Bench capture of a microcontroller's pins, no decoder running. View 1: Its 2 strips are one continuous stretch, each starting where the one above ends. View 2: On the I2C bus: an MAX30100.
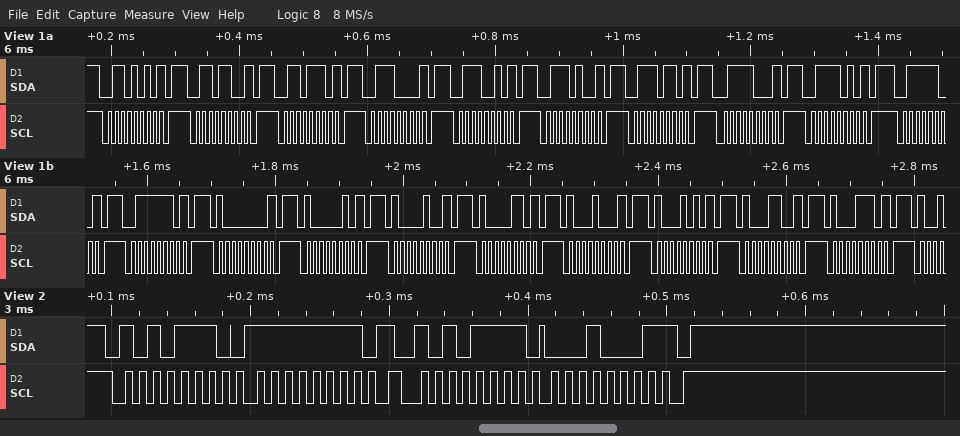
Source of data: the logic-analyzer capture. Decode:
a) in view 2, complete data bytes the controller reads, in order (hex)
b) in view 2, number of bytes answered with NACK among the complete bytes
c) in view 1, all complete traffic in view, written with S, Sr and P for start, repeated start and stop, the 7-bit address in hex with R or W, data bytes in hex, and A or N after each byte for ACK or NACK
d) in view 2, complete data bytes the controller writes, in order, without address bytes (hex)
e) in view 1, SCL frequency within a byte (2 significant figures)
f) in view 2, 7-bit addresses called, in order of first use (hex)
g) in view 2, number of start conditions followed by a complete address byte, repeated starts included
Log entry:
11
1
S 35W N P S 36W N P S 37W N P S 38W N P S 39W N P S 3AW N P S 3BW N P S 3CW N P S 3DW N P S 3EW N P S 3FW N P S 40W N P S 41W N P S 42W N P S 43W N P S 44W N P S 45W N P S 46W N P S 47W N P
FF
100 kHz
0x57
2
